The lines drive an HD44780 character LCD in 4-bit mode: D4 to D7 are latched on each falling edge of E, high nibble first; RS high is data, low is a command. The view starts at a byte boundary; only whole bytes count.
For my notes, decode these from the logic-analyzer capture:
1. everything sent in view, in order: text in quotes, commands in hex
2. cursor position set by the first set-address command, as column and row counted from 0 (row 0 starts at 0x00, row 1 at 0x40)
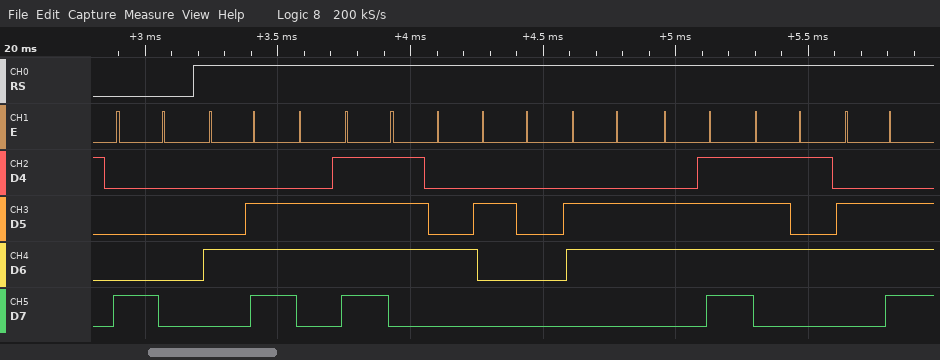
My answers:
0x80 "Not foun"
column 0, row 0
